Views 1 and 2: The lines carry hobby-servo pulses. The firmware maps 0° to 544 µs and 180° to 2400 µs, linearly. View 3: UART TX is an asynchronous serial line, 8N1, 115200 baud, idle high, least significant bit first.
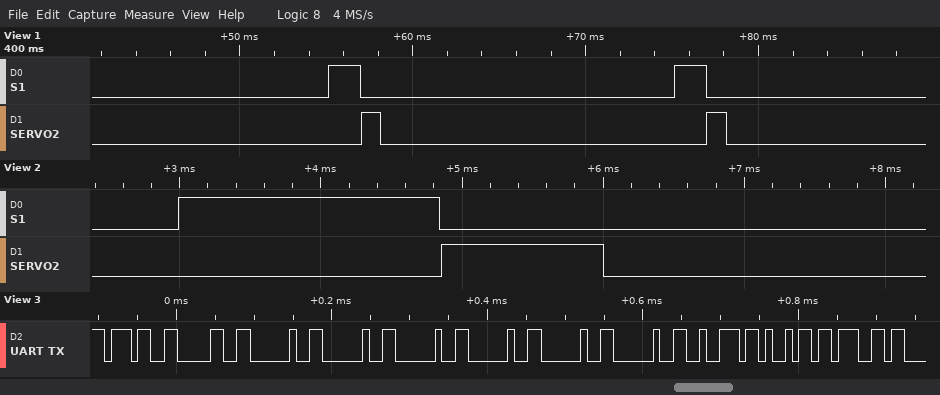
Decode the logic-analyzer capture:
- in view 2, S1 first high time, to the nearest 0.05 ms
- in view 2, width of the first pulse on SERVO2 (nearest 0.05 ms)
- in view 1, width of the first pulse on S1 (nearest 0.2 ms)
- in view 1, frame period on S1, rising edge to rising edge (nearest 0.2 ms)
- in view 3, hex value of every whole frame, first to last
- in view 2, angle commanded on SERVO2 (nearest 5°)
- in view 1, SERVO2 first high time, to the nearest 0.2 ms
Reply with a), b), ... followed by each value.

a) 1.85 ms
b) 1.15 ms
c) 1.8 ms
d) 20.0 ms
e) 37 30 20 20 20 20 20 20 72 69 67
f) 60°
g) 1.2 ms
